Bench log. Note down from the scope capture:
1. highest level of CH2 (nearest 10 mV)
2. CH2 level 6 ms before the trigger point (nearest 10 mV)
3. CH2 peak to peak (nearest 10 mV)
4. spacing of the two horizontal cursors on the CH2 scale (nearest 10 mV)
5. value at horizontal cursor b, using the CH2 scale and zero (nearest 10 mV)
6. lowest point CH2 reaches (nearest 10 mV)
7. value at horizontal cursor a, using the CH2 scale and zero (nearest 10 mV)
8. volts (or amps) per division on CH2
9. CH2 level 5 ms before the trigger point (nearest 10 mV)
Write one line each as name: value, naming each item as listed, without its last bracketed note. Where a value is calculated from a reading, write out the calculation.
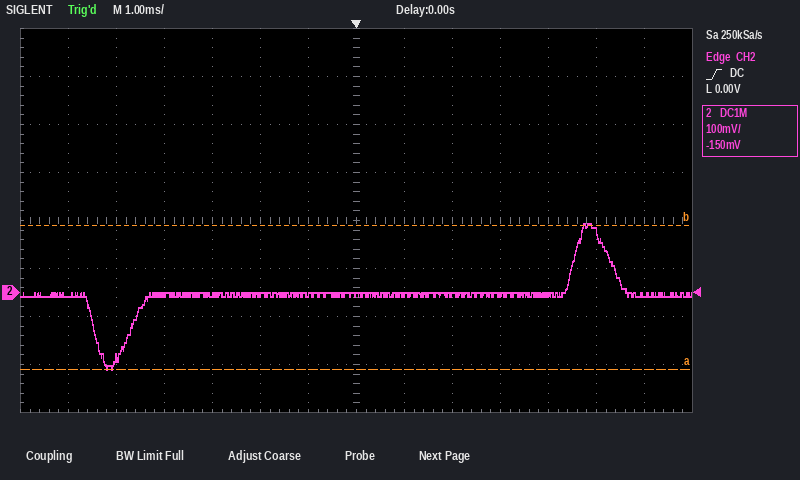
highest level of CH2: 140 mV
CH2 level 6 ms before the trigger point: -10 mV
CH2 peak to peak: 140 mV − (-160 mV) = 300 mV
spacing of the two horizontal cursors on the CH2 scale: 300 mV
value at horizontal cursor b, using the CH2 scale and zero: 140 mV
lowest point CH2 reaches: -160 mV
value at horizontal cursor a, using the CH2 scale and zero: -160 mV
volts (or amps) per division on CH2: 100 mV
CH2 level 5 ms before the trigger point: -140 mV
